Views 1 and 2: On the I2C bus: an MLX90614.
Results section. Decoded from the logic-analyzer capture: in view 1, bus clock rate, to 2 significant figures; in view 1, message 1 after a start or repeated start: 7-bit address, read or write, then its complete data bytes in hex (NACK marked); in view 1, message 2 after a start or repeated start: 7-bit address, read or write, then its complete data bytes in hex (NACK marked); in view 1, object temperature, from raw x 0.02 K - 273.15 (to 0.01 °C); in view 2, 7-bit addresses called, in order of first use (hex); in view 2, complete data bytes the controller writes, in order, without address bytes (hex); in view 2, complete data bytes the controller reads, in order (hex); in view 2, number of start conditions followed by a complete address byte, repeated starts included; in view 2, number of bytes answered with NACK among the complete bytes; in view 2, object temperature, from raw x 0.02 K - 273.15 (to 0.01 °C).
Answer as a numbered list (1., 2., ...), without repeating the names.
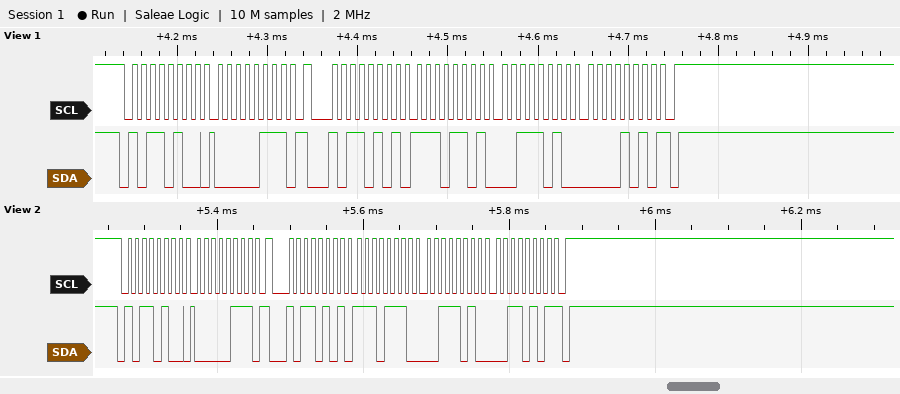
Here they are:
1. 100 kHz
2. 0x5A write: 07
3. 0x5A read: ED 3A 0A NACK
4. 28.55 °C
5. 0x5A
6. 07
7. EE 3A 35
8. 2
9. 1
10. 28.57 °C
